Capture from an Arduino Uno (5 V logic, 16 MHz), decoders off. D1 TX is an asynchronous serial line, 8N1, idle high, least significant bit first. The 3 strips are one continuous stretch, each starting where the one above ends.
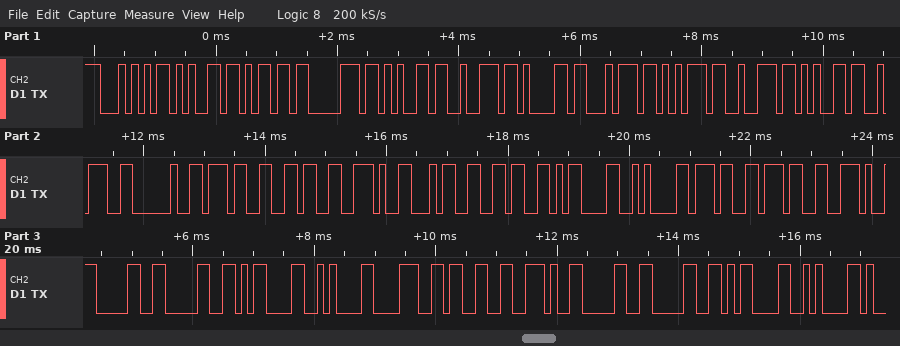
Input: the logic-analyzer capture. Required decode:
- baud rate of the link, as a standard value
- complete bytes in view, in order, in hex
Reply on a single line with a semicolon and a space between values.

9600 baud; 0x54 0x65 0x6D 0x70 0x65 0x72 0x61 0x74 0x75 0x72 0x65 0x3A 0x20 0x37 0x36 0x2E 0x34 0x36 0x0D 0x0A 0x37 0x37 0x2E 0x30 0x30 0x0D 0x0A 0x38 0x33 0x2E 0x30 0x30 0x0D 0x0A
